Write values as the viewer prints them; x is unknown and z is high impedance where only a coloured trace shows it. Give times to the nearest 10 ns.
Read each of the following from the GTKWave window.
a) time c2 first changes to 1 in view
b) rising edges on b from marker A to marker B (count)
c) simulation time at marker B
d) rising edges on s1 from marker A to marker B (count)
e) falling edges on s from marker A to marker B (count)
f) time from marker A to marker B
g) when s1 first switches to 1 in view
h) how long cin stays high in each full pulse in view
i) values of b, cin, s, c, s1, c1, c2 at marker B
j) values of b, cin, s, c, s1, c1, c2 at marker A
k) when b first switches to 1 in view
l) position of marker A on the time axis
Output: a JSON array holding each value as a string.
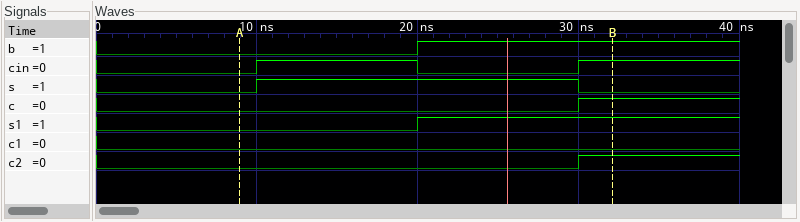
["30 ns", "1", "30 ns", "1", "1", "20 ns", "20 ns", "10 ns", "b=1, cin=1, s=0, c=1, s1=1, c1=0, c2=1", "b=0, cin=0, s=0, c=0, s1=0, c1=0, c2=0", "20 ns", "10 ns"]
